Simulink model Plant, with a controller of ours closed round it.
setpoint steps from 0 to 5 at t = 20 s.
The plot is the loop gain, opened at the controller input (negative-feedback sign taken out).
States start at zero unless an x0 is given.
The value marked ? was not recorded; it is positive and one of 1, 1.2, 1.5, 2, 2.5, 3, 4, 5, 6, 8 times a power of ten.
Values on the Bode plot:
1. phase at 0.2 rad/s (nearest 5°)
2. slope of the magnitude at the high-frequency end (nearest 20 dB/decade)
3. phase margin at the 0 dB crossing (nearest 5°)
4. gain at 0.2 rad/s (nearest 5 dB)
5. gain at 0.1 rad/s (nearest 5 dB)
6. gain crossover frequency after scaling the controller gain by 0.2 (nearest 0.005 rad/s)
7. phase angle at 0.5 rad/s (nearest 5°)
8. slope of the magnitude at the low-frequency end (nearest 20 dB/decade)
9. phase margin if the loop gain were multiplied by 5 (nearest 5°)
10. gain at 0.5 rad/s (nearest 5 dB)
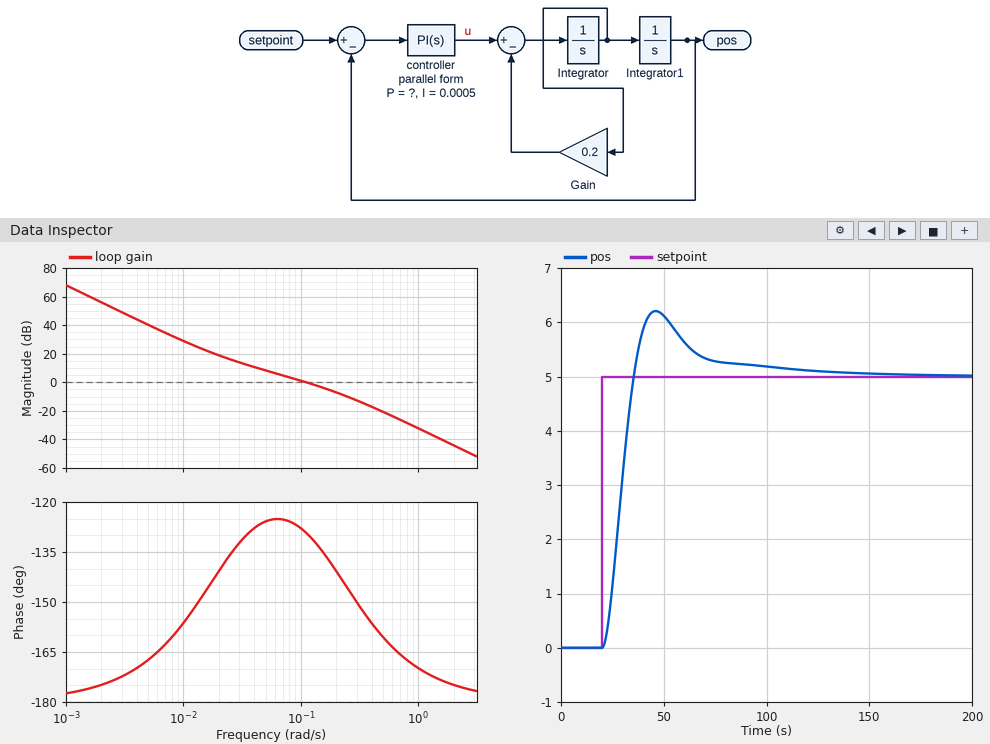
-140°
-40 dB/decade
50°
-5 dB
0 dB
0.030 rad/s
-160°
-40 dB/decade
30°
-20 dB
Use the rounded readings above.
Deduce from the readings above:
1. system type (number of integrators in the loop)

2
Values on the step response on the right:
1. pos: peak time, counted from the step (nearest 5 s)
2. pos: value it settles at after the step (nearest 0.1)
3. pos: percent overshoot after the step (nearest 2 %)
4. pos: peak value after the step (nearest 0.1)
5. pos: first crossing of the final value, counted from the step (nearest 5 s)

25 s
5.0
24 %
6.2
15 s
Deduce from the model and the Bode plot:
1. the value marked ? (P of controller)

0.025
